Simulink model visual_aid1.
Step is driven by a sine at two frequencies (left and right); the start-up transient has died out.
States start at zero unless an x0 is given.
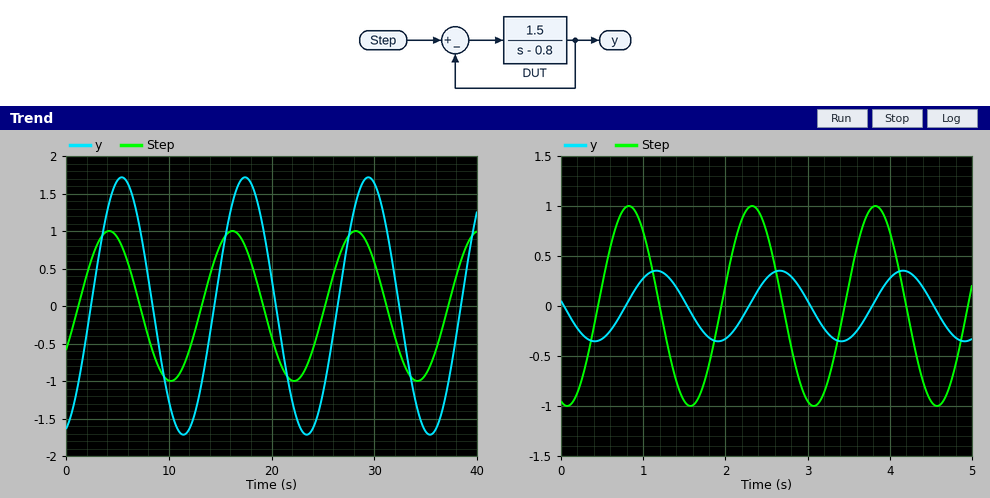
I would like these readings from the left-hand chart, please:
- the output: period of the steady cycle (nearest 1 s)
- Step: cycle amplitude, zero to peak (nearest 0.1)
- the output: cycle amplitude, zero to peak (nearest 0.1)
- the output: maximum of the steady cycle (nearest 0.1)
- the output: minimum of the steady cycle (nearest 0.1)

12 s
1.0
1.7
1.7
-1.7
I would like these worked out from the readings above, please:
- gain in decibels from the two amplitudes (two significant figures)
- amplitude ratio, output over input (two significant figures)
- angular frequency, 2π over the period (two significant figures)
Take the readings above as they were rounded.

4.6 dB
1.7
0.52 rad/s
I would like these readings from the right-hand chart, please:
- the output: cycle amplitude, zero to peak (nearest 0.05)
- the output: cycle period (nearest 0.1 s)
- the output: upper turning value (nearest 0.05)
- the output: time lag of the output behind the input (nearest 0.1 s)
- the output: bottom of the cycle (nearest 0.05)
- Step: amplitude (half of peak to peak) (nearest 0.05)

0.35
1.5 s
0.35
0.3 s
-0.35
1.00
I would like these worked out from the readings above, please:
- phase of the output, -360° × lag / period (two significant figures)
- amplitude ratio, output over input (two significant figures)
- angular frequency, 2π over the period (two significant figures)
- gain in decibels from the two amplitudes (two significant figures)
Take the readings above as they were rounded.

-72°
0.35
4.2 rad/s
-9.1 dB
